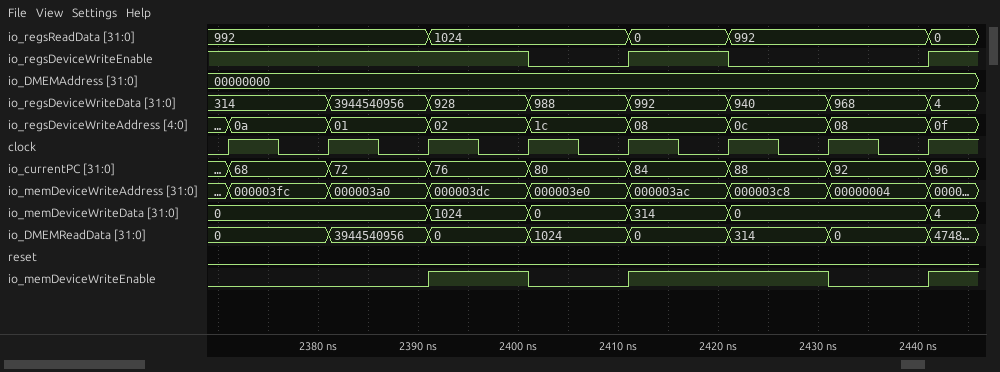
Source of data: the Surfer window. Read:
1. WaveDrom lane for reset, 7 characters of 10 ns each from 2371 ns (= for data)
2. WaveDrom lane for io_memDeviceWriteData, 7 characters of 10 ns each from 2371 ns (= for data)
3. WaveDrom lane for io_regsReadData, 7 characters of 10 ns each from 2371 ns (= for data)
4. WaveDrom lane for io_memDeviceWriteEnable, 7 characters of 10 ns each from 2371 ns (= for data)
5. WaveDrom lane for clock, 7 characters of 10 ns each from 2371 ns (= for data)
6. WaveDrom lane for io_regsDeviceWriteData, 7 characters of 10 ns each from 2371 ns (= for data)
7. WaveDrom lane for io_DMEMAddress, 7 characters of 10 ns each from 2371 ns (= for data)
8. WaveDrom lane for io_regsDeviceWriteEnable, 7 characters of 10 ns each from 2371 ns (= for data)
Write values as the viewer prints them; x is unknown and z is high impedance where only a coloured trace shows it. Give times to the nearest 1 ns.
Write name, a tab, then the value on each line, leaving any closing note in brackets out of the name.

WaveDrom lane for reset, 7 characters of 10 ns each from 2371 ns	{name: 'reset', wave: '0......'}
WaveDrom lane for io_memDeviceWriteData, 7 characters of 10 ns each from 2371 ns	{name: 'io_memDeviceWriteData', wave: '=.====.', data: '0 1024 0 314 0'}
WaveDrom lane for io_regsReadData, 7 characters of 10 ns each from 2371 ns	{name: 'io_regsReadData', wave: '=.=.==.', data: '992 1024 0 992'}
WaveDrom lane for io_memDeviceWriteEnable, 7 characters of 10 ns each from 2371 ns	{name: 'io_memDeviceWriteEnable', wave: '0.101.0'}
WaveDrom lane for clock, 7 characters of 10 ns each from 2371 ns	{name: 'clock', wave: 'p......'}
WaveDrom lane for io_regsDeviceWriteData, 7 characters of 10 ns each from 2371 ns	{name: 'io_regsDeviceWriteData', wave: '=======', data: '314 3944540956 928 988 992 940 968'}
WaveDrom lane for io_DMEMAddress, 7 characters of 10 ns each from 2371 ns	{name: 'io_DMEMAddress', wave: '=......', data: '00000000'}
WaveDrom lane for io_regsDeviceWriteEnable, 7 characters of 10 ns each from 2371 ns	{name: 'io_regsDeviceWriteEnable', wave: '1..010.'}
